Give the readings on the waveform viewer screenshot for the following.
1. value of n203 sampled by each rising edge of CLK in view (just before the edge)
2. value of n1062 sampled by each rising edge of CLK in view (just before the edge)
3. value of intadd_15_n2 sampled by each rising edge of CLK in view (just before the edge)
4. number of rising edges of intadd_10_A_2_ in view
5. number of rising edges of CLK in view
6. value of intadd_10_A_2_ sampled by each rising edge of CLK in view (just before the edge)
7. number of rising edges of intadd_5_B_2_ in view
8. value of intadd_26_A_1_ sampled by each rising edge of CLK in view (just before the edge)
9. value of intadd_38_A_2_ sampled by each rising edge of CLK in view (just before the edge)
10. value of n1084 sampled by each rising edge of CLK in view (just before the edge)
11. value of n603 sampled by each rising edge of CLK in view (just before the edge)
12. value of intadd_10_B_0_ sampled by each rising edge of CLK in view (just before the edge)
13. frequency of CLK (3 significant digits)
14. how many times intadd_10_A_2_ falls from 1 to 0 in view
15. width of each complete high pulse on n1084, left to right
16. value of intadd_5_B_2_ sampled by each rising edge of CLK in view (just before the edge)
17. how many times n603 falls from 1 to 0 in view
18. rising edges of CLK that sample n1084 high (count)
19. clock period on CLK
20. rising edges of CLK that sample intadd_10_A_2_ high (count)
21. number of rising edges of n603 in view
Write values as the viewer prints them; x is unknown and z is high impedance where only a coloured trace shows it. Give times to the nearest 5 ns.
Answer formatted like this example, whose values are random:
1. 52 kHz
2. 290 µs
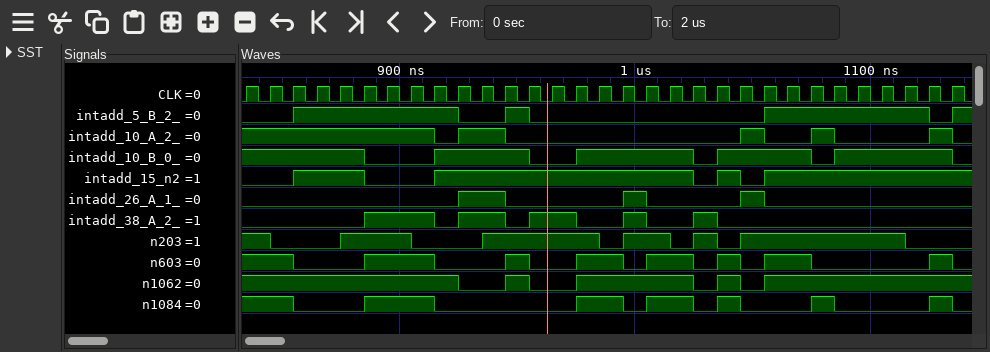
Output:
1. 1 1 0 0 0 1 1 1 0 0 0 1 1 1 1 1 0 1 1 0 1 0 1 1 1 1 1 1 1 0 0
2. 1 1 1 1 1 1 1 1 1 1 0 0 1 0 0 1 1 1 1 1 0 1 0 1 1 1 1 1 1 1 1
3. 0 0 0 1 1 1 0 0 0 1 1 1 1 1 1 1 1 1 1 1 0 1 0 1 1 1 1 1 1 1 1
4. 4
5. 31
6. 1 1 1 1 1 1 1 1 1 0 1 1 0 0 0 0 0 0 0 0 0 0 1 0 0 1 0 0 0 0 1
7. 4
8. 0 0 0 0 0 0 0 0 0 0 1 1 0 0 0 0 0 1 0 0 0 0 1 0 0 0 0 0 0 0 0
9. 0 0 0 0 0 0 1 1 1 0 1 1 0 1 1 0 0 1 0 0 1 0 0 0 0 0 0 0 0 0 0
10. 1 1 1 0 0 0 1 1 1 0 0 0 0 0 0 1 1 0 1 1 0 1 0 0 0 1 0 0 0 0 1
11. 1 1 1 0 0 0 1 1 1 0 0 0 1 0 0 1 1 0 1 1 0 1 0 1 1 0 0 0 0 0 1
12. 1 1 1 1 1 1 0 0 0 1 1 1 1 0 0 1 1 1 1 1 0 1 1 1 1 0 1 1 1 1 1
13. 100 MHz
14. 5
15. 30 ns, 20 ns, 20 ns, 10 ns, 10 ns, 10 ns
16. 0 0 0 1 1 1 1 1 1 1 0 0 1 0 0 0 0 0 0 0 0 0 0 1 1 1 1 1 1 1 0
17. 8
18. 13
19. 10 ns
20. 14
21. 7
